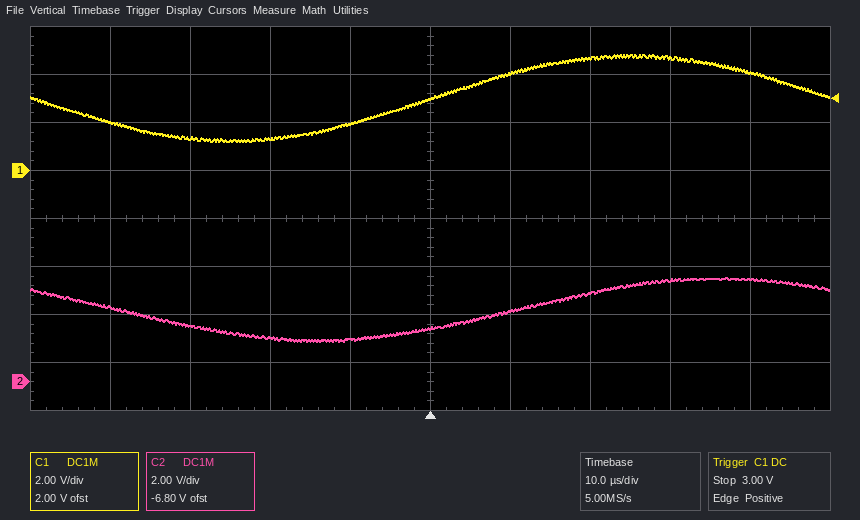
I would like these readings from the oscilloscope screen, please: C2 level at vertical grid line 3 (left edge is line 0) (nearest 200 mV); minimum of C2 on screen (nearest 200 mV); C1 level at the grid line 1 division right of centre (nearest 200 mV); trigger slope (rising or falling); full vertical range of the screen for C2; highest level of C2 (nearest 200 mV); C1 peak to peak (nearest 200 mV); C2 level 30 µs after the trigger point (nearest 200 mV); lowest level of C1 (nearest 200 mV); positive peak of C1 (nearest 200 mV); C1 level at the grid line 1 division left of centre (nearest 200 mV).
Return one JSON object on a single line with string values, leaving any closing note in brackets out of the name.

{"C2 level at vertical grid line 3 (left edge is line 0)": "1.8 V", "minimum of C2 on screen": "1.6 V", "C1 level at the grid line 1 division right of centre": "4.0 V", "trigger slope": "rising", "full vertical range of the screen for C2": "16 V", "highest level of C2": "4.4 V", "C1 peak to peak": "3.6 V", "C2 level 30 µs after the trigger point": "4.2 V", "lowest level of C1": "1.2 V", "positive peak of C1": "4.8 V", "C1 level at the grid line 1 division left of centre": "2.0 V"}
